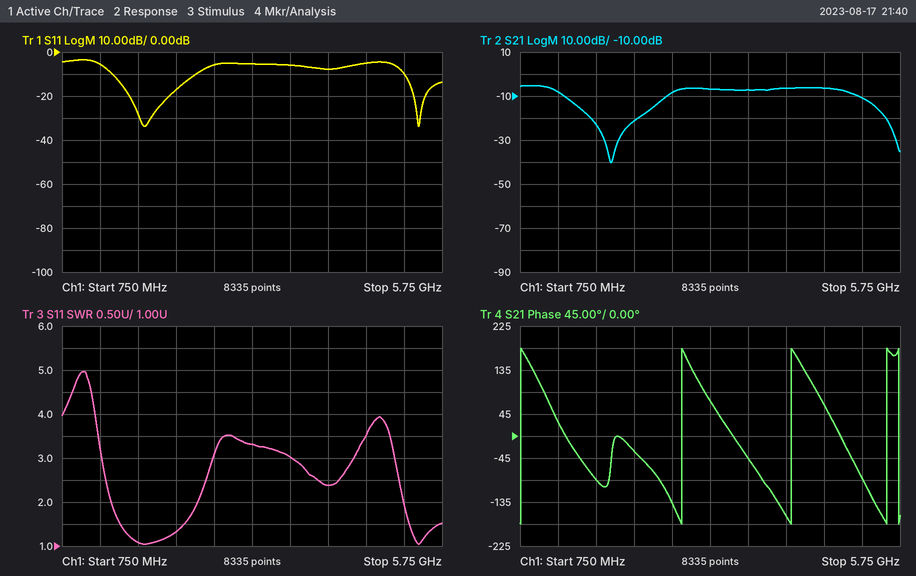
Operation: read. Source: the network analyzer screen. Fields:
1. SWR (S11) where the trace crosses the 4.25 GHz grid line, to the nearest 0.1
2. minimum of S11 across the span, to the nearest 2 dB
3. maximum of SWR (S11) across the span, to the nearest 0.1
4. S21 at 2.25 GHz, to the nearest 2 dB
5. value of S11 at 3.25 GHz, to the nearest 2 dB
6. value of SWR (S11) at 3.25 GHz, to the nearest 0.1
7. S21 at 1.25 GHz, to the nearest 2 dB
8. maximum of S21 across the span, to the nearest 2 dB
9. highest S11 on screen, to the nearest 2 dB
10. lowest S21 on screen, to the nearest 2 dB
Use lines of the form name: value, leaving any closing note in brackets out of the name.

SWR (S11) where the trace crosses the 4.25 GHz grid line, to the nearest 0.1: 2.4
minimum of S11 across the span, to the nearest 2 dB: -34 dB
maximum of SWR (S11) across the span, to the nearest 0.1: 5.0
S21 at 2.25 GHz, to the nearest 2 dB: -22 dB
value of S11 at 3.25 GHz, to the nearest 2 dB: -6 dB
value of SWR (S11) at 3.25 GHz, to the nearest 0.1: 3.3
S21 at 1.25 GHz, to the nearest 2 dB: -8 dB
maximum of S21 across the span, to the nearest 2 dB: -6 dB
highest S11 on screen, to the nearest 2 dB: -4 dB
lowest S21 on screen, to the nearest 2 dB: -40 dB
